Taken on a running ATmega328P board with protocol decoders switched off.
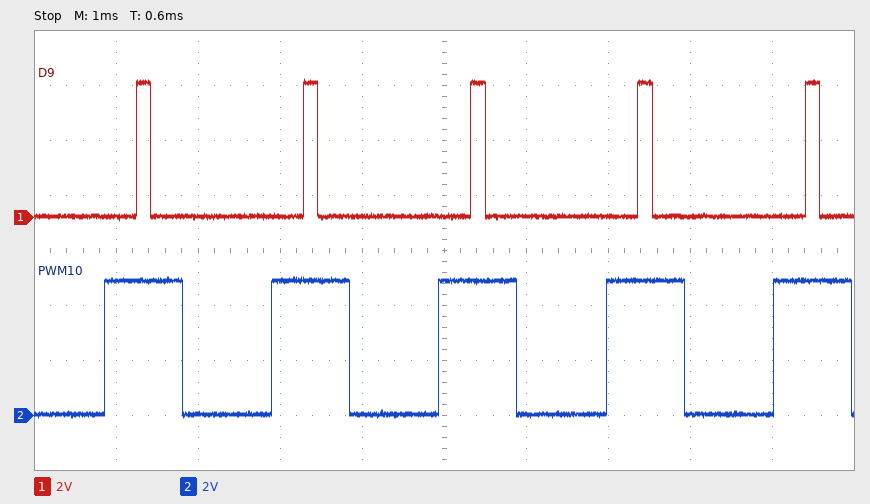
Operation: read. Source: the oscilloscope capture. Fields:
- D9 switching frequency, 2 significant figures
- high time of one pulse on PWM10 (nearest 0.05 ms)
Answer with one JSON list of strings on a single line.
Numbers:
["490 Hz", "0.95 ms"]
